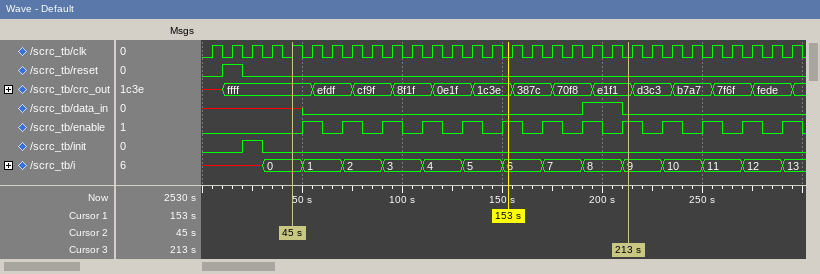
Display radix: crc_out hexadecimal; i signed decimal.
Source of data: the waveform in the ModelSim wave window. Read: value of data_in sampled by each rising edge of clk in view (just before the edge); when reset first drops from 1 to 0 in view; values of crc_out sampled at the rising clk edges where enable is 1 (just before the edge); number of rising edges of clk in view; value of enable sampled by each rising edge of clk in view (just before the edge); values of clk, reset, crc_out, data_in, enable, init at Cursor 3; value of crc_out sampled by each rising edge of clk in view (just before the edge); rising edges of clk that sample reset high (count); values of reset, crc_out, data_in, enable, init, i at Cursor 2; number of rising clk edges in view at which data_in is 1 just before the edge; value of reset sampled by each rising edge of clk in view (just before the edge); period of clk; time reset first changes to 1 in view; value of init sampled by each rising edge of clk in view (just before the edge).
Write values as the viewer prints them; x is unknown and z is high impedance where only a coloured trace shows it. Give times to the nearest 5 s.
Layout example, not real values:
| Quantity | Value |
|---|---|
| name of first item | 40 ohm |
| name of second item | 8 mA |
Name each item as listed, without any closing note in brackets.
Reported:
| Quantity | Value |
|---|---|
| value of data_in sampled by each rising edge of clk in view | x x x x x 0 0 0 0 0 0 0 0 0 0 0 0 0 0 1 1 0 0 0 0 0 0 0 0 0 |
| when reset first drops from 1 to 0 in view | 20 s |
| values of crc_out sampled at the rising clk edges where enable is 1 | ffff, efdf, cf9f, 8f1f, 0e1f, 1c3e, 387c, 70f8, e1f1, d3c3, b7a7, 7f6f, fede |
| number of rising edges of clk in view | 30 |
| value of enable sampled by each rising edge of clk in view | 0 0 0 0 0 1 0 1 0 1 0 1 0 1 0 1 0 1 0 1 0 1 0 1 0 1 0 1 0 1 |
| values of clk, reset, crc_out, data_in, enable, init at Cursor 3 | clk=0, reset=0, crc_out=e1f1, data_in=0, enable=1, init=0 |
| value of crc_out sampled by each rising edge of clk in view | x, ffff, ffff, ffff, ffff, ffff, efdf, efdf, cf9f, cf9f, 8f1f, 8f1f, 0e1f, 0e1f, 1c3e, 1c3e, 387c, 387c, 70f8, 70f8, e1f1, e1f1, d3c3, d3c3, b7a7, b7a7, 7f6f, 7f6f, fede, fede |
| rising edges of clk that sample reset high | 1 |
| values of reset, crc_out, data_in, enable, init, i at Cursor 2 | reset=0, crc_out=ffff, data_in=x, enable=0, init=0, i=0 |
| number of rising clk edges in view at which data_in is 1 just before the edge | 2 |
| value of reset sampled by each rising edge of clk in view | 0 1 0 0 0 0 0 0 0 0 0 0 0 0 0 0 0 0 0 0 0 0 0 0 0 0 0 0 0 0 |
| period of clk | 10 s |
| time reset first changes to 1 in view | 10 s |
| value of init sampled by each rising edge of clk in view | 0 0 1 0 0 0 0 0 0 0 0 0 0 0 0 0 0 0 0 0 0 0 0 0 0 0 0 0 0 0 |
